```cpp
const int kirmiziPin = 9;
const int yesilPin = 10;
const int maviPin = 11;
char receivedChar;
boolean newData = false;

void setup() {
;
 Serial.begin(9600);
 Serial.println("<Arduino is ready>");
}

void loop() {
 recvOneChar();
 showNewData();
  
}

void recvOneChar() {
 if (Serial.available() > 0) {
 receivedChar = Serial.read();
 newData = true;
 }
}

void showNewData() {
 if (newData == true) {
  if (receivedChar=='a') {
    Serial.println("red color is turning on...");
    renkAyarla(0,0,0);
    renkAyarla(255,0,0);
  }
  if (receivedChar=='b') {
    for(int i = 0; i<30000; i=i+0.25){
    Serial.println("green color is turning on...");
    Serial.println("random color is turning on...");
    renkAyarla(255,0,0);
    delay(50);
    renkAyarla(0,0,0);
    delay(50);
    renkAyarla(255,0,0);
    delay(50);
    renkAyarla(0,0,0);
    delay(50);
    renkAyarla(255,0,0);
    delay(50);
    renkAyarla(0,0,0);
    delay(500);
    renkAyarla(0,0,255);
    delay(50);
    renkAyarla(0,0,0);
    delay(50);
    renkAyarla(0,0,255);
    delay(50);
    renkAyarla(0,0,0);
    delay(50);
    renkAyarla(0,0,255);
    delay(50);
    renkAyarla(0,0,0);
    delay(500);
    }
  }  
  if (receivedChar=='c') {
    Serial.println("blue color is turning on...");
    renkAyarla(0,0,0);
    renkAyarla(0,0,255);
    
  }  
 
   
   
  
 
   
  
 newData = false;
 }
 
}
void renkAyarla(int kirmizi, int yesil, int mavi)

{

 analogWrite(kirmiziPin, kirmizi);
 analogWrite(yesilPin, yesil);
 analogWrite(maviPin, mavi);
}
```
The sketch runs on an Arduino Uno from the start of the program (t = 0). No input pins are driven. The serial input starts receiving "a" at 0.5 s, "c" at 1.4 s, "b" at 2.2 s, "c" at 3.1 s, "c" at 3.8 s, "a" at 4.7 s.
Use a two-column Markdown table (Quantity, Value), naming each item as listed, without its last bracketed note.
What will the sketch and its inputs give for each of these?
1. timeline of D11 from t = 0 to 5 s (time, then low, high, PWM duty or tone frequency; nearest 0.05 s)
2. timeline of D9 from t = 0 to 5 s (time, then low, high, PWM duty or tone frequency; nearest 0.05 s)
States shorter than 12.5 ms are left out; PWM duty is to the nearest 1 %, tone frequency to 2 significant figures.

| Quantity | Value |
|---|---|
| timeline of D11 from t = 0 to 5 s | 0.5 s low; 1.4 s high; 2.2 s low; 2.95 s high; 3 s low; 3.05 s high; 3.1 s low; 3.15 s high; 3.2 s low; 4.45 s high; 4.5 s low; 4.55 s high; 4.6 s low; 4.65 s high; 4.7 s low |
| timeline of D9 from t = 0 to 5 s | 0.5 s high; 1.4 s low; 2.2 s high; 2.25 s low; 2.3 s high; 2.35 s low; 2.4 s high; 2.45 s low; 3.7 s high; 3.75 s low; 3.8 s high; 3.85 s low; 3.9 s high; 3.95 s low |
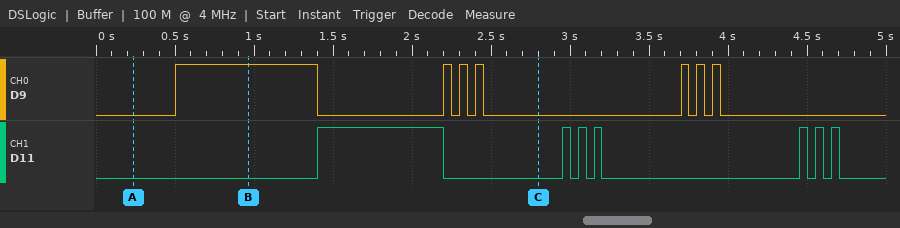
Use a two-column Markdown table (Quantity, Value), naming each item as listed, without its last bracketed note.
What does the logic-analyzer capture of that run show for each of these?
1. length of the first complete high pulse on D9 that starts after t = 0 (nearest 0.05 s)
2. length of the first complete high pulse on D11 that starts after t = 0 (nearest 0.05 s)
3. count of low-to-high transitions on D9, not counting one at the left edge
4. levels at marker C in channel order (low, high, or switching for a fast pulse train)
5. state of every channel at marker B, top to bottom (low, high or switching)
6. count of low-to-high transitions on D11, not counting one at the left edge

| Quantity | Value |
|---|---|
| length of the first complete high pulse on D9 that starts after t = 0 | 0.90 s |
| length of the first complete high pulse on D11 that starts after t = 0 | 0.80 s |
| count of low-to-high transitions on D9, not counting one at the left edge | 7 |
| levels at marker C in channel order | D9 low, D11 low |
| state of every channel at marker B, top to bottom | D9 high, D11 low |
| count of low-to-high transitions on D11, not counting one at the left edge | 7 |
